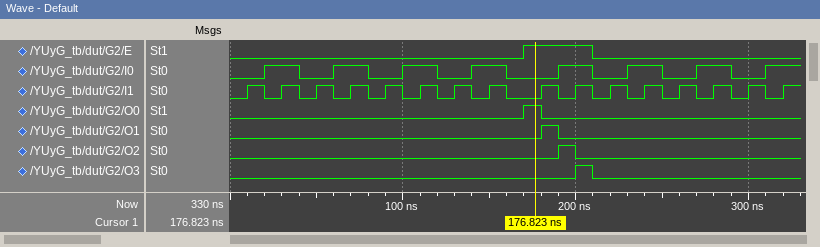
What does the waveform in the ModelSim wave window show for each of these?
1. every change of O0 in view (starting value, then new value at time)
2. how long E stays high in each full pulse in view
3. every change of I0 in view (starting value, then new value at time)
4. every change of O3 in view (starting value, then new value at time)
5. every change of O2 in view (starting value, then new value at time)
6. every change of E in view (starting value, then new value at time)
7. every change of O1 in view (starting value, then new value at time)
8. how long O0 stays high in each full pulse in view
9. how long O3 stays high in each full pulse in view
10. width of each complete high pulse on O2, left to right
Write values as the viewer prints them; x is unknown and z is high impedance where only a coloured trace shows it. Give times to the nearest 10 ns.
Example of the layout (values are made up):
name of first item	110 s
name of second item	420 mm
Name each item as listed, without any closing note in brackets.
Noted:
every change of O0 in view	0, 1 at 170 ns, 0 at 180 ns
how long E stays high in each full pulse in view	40 ns
every change of I0 in view	0, 1 at 20 ns, 0 at 40 ns, 1 at 60 ns, 0 at 80 ns, 1 at 100 ns, 0 at 120 ns, 1 at 140 ns, 0 at 160 ns, 1 at 190 ns, 0 at 210 ns, 1 at 230 ns, 0 at 250 ns, 1 at 270 ns, 0 at 290 ns, 1 at 310 ns
every change of O3 in view	0, 1 at 200 ns, 0 at 210 ns
every change of O2 in view	0, 1 at 190 ns, 0 at 200 ns
every change of E in view	0, 1 at 170 ns, 0 at 210 ns
every change of O1 in view	0, 1 at 180 ns, 0 at 190 ns
how long O0 stays high in each full pulse in view	10 ns
how long O3 stays high in each full pulse in view	10 ns
width of each complete high pulse on O2, left to right	10 ns
